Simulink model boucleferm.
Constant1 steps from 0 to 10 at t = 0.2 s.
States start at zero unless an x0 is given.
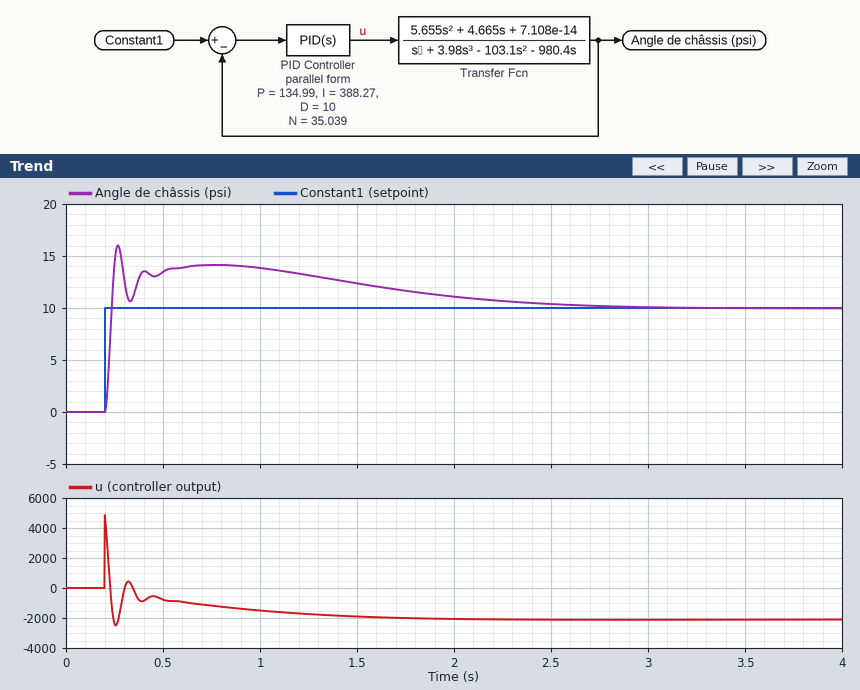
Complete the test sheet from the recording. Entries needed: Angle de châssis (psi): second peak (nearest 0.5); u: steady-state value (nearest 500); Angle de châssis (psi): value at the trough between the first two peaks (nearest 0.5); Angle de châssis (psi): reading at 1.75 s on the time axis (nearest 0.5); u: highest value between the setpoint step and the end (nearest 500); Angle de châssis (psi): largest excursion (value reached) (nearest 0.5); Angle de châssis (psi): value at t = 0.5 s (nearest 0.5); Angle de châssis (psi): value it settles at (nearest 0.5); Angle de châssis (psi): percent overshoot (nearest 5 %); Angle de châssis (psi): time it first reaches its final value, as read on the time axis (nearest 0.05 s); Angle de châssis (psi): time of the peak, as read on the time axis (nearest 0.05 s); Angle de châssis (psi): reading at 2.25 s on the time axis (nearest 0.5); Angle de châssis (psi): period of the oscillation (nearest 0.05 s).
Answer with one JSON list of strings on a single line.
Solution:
["14.0", "-2000", "10.5", "11.5", "5000", "16.0", "13.5", "10.0", "60 %", "0.25 s", "0.25 s", "10.5", "0.50 s"]
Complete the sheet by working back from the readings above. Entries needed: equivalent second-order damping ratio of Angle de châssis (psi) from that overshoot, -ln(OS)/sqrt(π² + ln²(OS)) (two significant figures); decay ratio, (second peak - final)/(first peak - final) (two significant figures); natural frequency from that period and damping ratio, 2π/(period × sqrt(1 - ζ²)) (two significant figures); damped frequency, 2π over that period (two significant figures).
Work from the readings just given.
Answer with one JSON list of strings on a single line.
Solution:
["0.16", "0.67", "13 rad/s", "13 rad/s"]
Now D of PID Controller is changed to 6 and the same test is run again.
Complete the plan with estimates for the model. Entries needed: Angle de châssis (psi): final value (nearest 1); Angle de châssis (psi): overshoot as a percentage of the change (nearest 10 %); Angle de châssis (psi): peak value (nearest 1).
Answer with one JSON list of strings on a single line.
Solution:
["10", "70 %", "17"]
